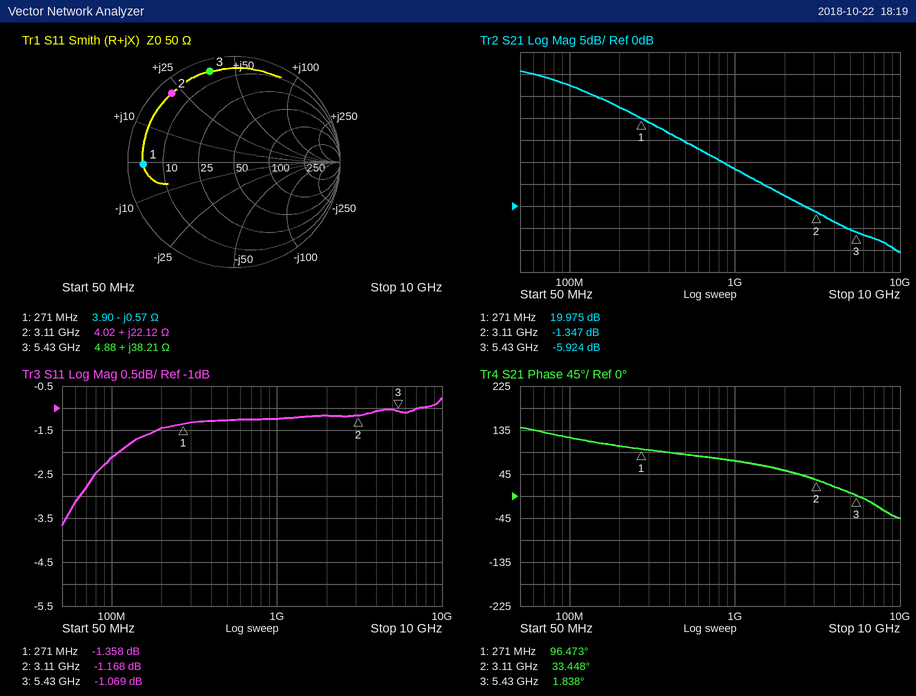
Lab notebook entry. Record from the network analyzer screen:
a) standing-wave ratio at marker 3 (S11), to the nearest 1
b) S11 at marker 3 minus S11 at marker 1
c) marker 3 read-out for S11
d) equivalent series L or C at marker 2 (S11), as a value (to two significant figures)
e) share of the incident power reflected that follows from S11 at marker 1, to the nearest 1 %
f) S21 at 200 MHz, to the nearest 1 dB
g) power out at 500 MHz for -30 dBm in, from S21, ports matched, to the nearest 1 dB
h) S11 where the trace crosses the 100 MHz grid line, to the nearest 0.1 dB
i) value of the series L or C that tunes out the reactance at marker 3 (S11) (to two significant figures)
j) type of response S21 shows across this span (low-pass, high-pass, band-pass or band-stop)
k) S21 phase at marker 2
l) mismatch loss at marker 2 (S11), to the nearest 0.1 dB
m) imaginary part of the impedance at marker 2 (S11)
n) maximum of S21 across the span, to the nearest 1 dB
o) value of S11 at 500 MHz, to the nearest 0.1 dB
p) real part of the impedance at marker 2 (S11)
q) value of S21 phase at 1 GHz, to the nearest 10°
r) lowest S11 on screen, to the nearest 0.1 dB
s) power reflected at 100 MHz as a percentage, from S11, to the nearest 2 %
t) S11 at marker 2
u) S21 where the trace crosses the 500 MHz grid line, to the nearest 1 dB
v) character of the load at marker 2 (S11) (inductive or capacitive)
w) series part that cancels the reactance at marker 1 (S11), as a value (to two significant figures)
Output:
16
0.289 dB
-1.069 dB
1.1 nH
73 %
22 dB
-15 dBm
-2.1 dB
770 fF
low-pass
33.448°
6.3 dB
+22.12 Ω
31 dB
-1.3 dB
4.02 Ω
70°
-3.7 dB
62 %
-1.168 dB
15 dB
inductive
330 pH
